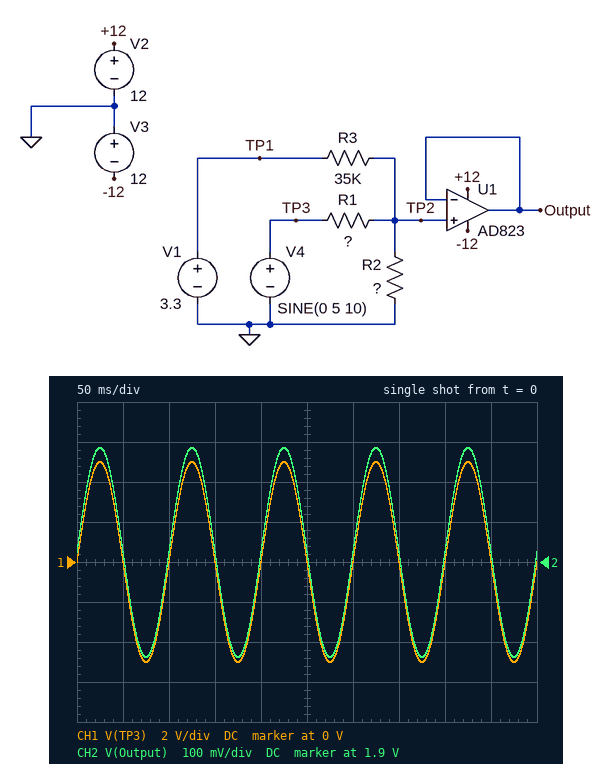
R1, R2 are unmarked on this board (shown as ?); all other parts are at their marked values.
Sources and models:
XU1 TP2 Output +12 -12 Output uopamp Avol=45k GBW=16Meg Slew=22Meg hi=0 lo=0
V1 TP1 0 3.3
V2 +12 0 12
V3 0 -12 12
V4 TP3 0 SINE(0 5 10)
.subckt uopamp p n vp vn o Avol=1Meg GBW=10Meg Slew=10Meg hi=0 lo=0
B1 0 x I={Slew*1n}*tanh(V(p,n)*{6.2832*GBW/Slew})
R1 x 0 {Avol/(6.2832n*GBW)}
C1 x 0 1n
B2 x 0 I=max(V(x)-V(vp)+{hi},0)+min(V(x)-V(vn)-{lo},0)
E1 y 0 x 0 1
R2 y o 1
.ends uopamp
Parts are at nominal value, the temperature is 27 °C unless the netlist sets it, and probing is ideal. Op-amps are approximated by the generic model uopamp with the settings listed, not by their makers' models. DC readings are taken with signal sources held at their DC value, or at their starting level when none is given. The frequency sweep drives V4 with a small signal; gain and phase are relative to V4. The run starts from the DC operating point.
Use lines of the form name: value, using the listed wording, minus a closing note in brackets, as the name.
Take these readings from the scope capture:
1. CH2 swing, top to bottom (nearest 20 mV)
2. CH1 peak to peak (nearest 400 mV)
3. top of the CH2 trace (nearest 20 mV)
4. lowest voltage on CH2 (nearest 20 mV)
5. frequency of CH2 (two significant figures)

CH2 swing, top to bottom: 520 mV
CH1 peak to peak: 10.0 V
top of the CH2 trace: 2.18 V
lowest voltage on CH2: 1.66 V
frequency of CH2: 10 Hz
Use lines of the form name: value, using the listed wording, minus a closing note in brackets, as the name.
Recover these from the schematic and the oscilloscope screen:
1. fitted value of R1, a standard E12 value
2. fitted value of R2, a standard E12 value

fitted value of R1, a standard E12 value: 390 kΩ
fitted value of R2, a standard E12 value: 56 kΩ
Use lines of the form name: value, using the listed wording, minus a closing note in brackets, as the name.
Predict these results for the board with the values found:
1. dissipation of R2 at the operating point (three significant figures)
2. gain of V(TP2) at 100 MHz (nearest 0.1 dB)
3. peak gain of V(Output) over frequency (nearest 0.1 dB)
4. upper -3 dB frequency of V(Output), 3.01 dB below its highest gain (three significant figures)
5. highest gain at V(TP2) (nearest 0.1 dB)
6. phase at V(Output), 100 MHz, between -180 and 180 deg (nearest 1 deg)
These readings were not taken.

dissipation of R2 at the operating point: 66.1 µW
gain of V(TP2) at 100 MHz: -25.6 dB
peak gain of V(Output) over frequency: -25.6 dB
upper -3 dB frequency of V(Output), 3.01 dB below its highest gain: 16.0 MHz
highest gain at V(TP2): -25.6 dB
phase at V(Output), 100 MHz, between -180 and 180 deg: -81 deg
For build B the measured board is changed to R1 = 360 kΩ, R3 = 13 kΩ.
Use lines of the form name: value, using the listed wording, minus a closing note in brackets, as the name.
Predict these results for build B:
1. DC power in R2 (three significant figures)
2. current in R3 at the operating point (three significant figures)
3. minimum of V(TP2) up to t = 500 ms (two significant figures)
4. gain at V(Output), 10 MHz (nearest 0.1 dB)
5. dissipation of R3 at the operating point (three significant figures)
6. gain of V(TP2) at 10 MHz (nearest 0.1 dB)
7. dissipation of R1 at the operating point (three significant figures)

DC power in R2: 121 µW
current in R3 at the operating point: 53.7 µA
minimum of V(TP2) up to t = 500 ms: 2.5 V
gain at V(Output), 10 MHz: -32.3 dB
dissipation of R3 at the operating point: 37.5 µW
gain of V(TP2) at 10 MHz: -30.9 dB
dissipation of R1 at the operating point: 18.8 µW
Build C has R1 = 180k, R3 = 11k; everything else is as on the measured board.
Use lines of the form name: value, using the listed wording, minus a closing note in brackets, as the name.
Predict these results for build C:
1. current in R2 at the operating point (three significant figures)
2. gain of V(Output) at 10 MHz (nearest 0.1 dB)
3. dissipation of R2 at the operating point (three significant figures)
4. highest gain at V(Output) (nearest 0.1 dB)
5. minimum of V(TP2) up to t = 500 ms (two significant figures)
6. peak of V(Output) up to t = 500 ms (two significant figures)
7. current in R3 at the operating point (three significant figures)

current in R2 at the operating point: 46.9 µA
gain of V(Output) at 10 MHz: -27.7 dB
dissipation of R2 at the operating point: 123 µW
highest gain at V(Output): -26.3 dB
minimum of V(TP2) up to t = 500 ms: 2.4 V
peak of V(Output) up to t = 500 ms: 2.9 V
current in R3 at the operating point: 61.4 µA
